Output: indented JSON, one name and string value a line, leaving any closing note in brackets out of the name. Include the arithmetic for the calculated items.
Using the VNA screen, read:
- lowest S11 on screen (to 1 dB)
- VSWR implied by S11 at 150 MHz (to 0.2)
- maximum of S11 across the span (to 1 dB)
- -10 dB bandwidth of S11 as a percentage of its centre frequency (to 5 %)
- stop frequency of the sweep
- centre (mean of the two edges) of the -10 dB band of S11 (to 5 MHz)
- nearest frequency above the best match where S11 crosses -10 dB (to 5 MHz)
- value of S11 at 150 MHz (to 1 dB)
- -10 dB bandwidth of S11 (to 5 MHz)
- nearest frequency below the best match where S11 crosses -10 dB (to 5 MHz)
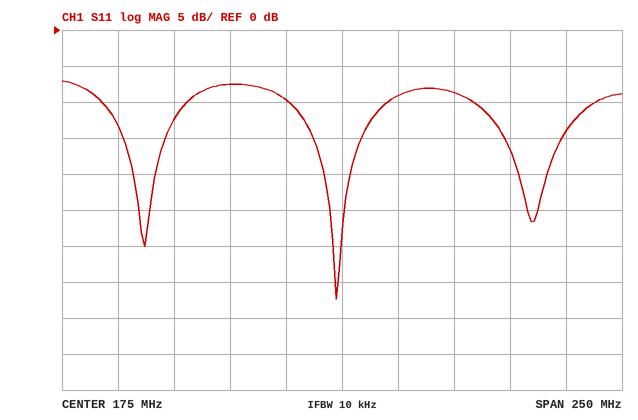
{
  "lowest S11 on screen": "-37 dB",
  "VSWR implied by S11 at 150 MHz": "|Γ| = 10^(-10/20) = 0.3162; VSWR = (1 + 0.3162)/(1 − 0.3162) ≈ 1.92, so 2.0 to the nearest 0.2",
  "maximum of S11 across the span": "-7 dB",
  "-10 dB bandwidth of S11 as a percentage of its centre frequency": "45 MHz / 172.5 MHz ≈ 26.1 %, so 25 % to the nearest 5 %",
  "stop frequency of the sweep": "300 MHz",
  "centre (mean of the two edges) of the -10 dB band of S11": "175 MHz",
  "nearest frequency above the best match where S11 crosses -10 dB": "195 MHz",
  "value of S11 at 150 MHz": "-10 dB",
  "-10 dB bandwidth of S11": "195 MHz − 150 MHz = 45 MHz",
  "nearest frequency below the best match where S11 crosses -10 dB": "150 MHz"
}
